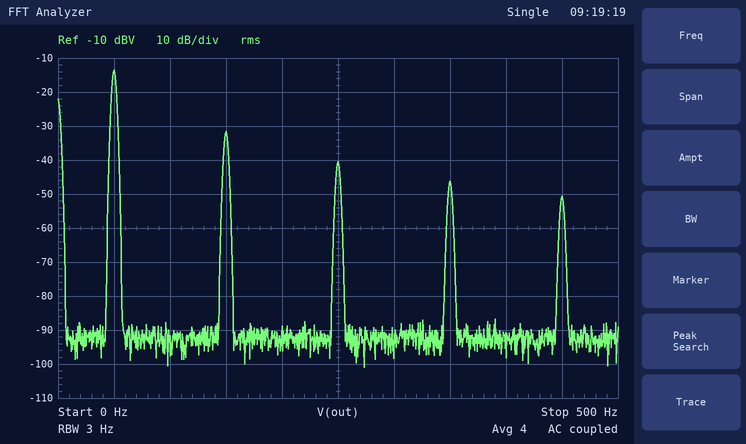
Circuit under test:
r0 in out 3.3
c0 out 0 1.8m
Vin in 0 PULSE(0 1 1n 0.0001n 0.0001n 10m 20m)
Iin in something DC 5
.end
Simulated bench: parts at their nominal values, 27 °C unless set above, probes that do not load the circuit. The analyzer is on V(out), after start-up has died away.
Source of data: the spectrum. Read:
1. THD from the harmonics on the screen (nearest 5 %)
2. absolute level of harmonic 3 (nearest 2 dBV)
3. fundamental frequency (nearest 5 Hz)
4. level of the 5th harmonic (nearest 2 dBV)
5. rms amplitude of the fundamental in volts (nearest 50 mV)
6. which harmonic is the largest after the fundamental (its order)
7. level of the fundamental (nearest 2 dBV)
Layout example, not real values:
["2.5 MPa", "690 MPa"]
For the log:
["15 %", "-32 dBV", "50 Hz", "-40 dBV", "200 mV", "3", "-14 dBV"]
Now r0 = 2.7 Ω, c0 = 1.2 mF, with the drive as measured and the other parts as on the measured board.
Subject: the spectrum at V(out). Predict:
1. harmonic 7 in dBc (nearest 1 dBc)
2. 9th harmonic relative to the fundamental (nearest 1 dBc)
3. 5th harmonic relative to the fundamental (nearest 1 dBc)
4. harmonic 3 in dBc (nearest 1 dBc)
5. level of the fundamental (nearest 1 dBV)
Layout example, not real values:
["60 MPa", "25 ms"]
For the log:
["-31 dBc", "-35 dBc", "-25 dBc", "-17 dBc", "-10 dBV"]
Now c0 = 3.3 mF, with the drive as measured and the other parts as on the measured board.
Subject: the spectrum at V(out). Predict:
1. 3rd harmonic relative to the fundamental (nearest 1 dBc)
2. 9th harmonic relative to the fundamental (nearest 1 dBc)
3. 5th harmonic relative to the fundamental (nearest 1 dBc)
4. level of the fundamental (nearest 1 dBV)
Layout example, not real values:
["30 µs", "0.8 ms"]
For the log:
["-19 dBc", "-38 dBc", "-28 dBc", "-18 dBV"]
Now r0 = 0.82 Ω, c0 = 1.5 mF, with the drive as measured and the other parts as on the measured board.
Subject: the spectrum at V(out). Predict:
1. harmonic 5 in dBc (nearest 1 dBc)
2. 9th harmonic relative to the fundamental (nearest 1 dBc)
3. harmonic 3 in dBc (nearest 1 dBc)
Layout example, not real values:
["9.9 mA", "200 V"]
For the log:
["-20 dBc", "-30 dBc", "-13 dBc"]
